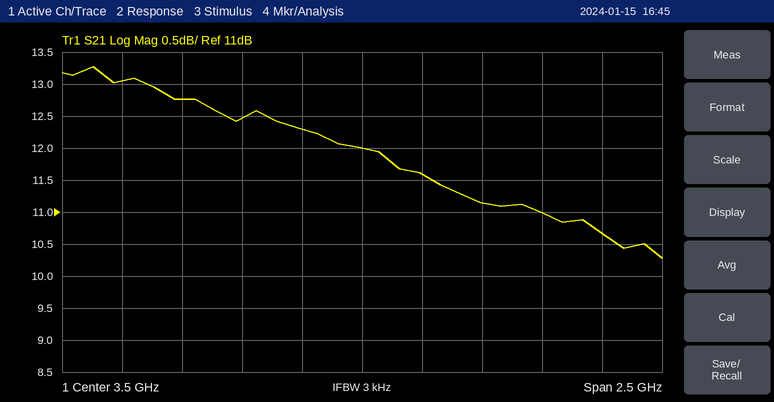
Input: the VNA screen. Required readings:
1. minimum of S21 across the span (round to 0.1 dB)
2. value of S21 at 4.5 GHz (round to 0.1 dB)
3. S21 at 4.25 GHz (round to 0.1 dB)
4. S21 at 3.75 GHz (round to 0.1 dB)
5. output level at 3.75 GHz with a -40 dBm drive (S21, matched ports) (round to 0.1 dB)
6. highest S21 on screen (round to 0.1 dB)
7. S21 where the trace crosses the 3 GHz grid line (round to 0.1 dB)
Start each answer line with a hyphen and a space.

- 10.3 dB
- 10.7 dB
- 11.0 dB
- 11.6 dB
- -28.4 dBm
- 13.3 dB
- 12.5 dB
